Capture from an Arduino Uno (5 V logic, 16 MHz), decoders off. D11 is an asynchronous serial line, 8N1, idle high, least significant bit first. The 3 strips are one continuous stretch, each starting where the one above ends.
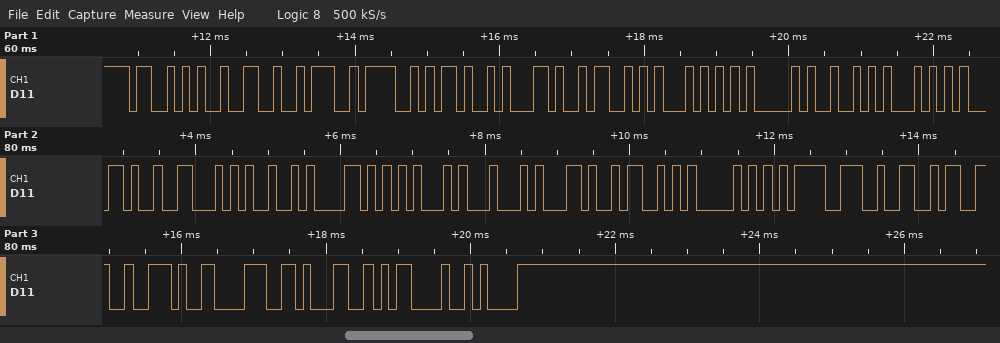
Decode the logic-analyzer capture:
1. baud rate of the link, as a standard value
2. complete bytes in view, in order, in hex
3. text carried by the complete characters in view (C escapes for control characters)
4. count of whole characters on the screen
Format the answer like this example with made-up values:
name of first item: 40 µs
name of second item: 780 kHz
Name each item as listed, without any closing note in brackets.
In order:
baud rate of the link, as a standard value: 9600 baud
complete bytes in view, in order, in hex: 53 32 3A 4F 4B 2C 53 54 41 52 54 2C 46 49 58 45 44 2C 53 50 3D 32 33 2E 38 31 0D 0A
text carried by the complete characters in view: "S2:OK,START,FIXED,SP=23.81\r\n"
count of whole characters on the screen: 28
